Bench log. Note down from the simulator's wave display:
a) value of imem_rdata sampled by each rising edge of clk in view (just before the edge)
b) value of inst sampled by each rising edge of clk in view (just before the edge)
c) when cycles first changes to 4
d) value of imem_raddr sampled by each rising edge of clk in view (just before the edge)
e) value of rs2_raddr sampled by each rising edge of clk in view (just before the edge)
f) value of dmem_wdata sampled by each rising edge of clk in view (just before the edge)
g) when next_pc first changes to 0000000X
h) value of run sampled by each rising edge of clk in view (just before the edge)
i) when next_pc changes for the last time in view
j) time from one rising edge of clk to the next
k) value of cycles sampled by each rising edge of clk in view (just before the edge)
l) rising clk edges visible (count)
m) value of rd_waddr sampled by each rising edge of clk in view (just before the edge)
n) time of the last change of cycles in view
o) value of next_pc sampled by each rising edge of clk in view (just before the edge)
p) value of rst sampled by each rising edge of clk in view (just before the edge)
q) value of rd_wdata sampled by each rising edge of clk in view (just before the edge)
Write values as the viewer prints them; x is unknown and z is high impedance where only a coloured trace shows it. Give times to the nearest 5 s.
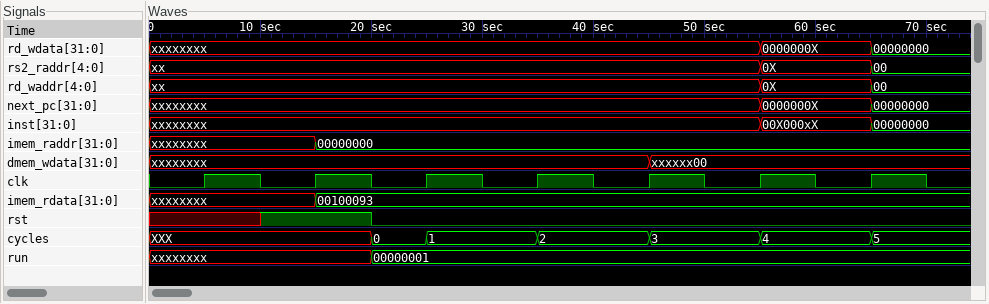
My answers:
xxxxxxxx, xxxxxxxx, 00100093, 00100093, 00100093, 00100093, 00100093
xxxxxxxx, xxxxxxxx, xxxxxxxx, xxxxxxxx, xxxxxxxx, xxxxxxxx, 00X000xX
55 s
xxxxxxxx, xxxxxxxx, 00000000, 00000000, 00000000, 00000000, 00000000
xx, xx, xx, xx, xx, xx, 0X
xxxxxxxx, xxxxxxxx, xxxxxxxx, xxxxxxxx, xxxxxxxx, xxxxxx00, xxxxxx00
55 s
xxxxxxxx, xxxxxxxx, 00000001, 00000001, 00000001, 00000001, 00000001
65 s
10 s
XXX, XXX, 0, 1, 2, 3, 4
7
xx, xx, xx, xx, xx, xx, 0X
65 s
xxxxxxxx, xxxxxxxx, xxxxxxxx, xxxxxxxx, xxxxxxxx, xxxxxxxx, 0000000X
x 1 0 0 0 0 0
xxxxxxxx, xxxxxxxx, xxxxxxxx, xxxxxxxx, xxxxxxxx, xxxxxxxx, 0000000X
